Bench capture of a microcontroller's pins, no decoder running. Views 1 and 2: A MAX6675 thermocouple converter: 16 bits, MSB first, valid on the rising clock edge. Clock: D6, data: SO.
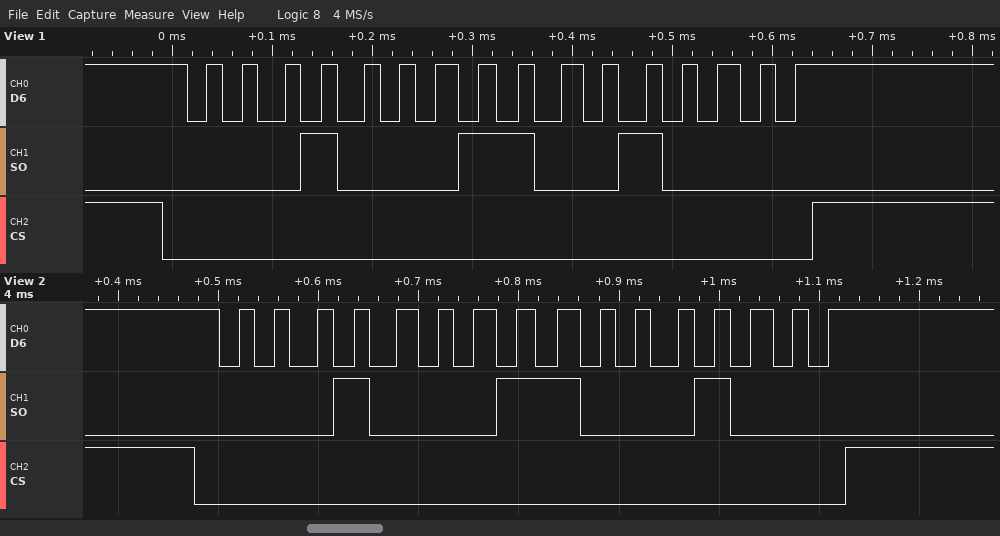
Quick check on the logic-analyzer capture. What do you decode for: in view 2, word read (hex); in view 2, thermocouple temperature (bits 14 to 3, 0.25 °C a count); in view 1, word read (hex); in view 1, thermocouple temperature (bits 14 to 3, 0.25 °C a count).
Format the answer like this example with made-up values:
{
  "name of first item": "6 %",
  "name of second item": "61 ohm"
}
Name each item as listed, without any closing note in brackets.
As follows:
{
  "in view 2, word read": "0x1188",
  "in view 2, thermocouple temperature": "140.25 °C",
  "in view 1, word read": "0x1190",
  "in view 1, thermocouple temperature": "140.50 °C"
}
